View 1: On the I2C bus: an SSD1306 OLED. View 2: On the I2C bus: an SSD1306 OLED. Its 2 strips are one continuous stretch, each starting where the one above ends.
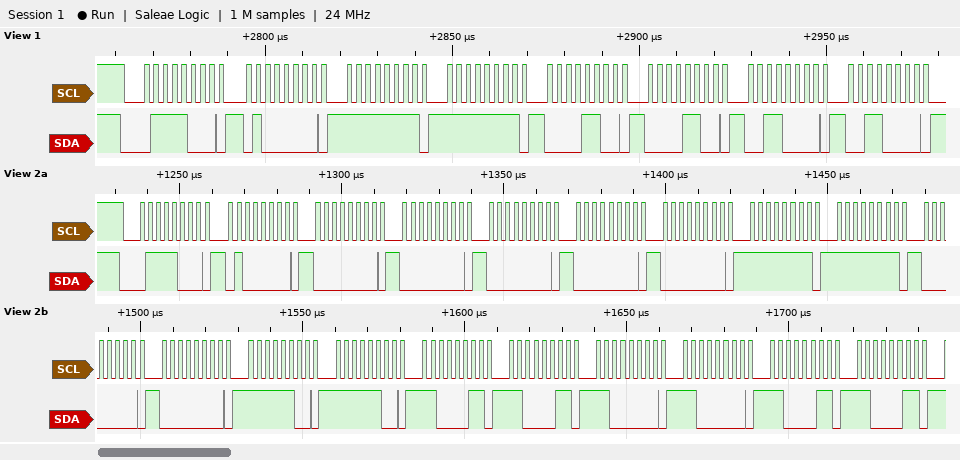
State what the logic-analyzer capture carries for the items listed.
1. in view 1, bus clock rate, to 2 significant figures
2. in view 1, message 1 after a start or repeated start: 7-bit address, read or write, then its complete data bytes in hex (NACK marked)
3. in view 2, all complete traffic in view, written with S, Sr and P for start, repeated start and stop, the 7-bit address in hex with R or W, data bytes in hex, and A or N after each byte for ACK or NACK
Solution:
400 kHz
0x3C write: 40 FF FF 0C 0C 30 30
S 3CW A 40 A 00 A 00 A 00 A 00 A 00 A FF A FF A 00 A 00 A FC A FC A C3 A C3 A C0 A C0 A C3 A C3 A
